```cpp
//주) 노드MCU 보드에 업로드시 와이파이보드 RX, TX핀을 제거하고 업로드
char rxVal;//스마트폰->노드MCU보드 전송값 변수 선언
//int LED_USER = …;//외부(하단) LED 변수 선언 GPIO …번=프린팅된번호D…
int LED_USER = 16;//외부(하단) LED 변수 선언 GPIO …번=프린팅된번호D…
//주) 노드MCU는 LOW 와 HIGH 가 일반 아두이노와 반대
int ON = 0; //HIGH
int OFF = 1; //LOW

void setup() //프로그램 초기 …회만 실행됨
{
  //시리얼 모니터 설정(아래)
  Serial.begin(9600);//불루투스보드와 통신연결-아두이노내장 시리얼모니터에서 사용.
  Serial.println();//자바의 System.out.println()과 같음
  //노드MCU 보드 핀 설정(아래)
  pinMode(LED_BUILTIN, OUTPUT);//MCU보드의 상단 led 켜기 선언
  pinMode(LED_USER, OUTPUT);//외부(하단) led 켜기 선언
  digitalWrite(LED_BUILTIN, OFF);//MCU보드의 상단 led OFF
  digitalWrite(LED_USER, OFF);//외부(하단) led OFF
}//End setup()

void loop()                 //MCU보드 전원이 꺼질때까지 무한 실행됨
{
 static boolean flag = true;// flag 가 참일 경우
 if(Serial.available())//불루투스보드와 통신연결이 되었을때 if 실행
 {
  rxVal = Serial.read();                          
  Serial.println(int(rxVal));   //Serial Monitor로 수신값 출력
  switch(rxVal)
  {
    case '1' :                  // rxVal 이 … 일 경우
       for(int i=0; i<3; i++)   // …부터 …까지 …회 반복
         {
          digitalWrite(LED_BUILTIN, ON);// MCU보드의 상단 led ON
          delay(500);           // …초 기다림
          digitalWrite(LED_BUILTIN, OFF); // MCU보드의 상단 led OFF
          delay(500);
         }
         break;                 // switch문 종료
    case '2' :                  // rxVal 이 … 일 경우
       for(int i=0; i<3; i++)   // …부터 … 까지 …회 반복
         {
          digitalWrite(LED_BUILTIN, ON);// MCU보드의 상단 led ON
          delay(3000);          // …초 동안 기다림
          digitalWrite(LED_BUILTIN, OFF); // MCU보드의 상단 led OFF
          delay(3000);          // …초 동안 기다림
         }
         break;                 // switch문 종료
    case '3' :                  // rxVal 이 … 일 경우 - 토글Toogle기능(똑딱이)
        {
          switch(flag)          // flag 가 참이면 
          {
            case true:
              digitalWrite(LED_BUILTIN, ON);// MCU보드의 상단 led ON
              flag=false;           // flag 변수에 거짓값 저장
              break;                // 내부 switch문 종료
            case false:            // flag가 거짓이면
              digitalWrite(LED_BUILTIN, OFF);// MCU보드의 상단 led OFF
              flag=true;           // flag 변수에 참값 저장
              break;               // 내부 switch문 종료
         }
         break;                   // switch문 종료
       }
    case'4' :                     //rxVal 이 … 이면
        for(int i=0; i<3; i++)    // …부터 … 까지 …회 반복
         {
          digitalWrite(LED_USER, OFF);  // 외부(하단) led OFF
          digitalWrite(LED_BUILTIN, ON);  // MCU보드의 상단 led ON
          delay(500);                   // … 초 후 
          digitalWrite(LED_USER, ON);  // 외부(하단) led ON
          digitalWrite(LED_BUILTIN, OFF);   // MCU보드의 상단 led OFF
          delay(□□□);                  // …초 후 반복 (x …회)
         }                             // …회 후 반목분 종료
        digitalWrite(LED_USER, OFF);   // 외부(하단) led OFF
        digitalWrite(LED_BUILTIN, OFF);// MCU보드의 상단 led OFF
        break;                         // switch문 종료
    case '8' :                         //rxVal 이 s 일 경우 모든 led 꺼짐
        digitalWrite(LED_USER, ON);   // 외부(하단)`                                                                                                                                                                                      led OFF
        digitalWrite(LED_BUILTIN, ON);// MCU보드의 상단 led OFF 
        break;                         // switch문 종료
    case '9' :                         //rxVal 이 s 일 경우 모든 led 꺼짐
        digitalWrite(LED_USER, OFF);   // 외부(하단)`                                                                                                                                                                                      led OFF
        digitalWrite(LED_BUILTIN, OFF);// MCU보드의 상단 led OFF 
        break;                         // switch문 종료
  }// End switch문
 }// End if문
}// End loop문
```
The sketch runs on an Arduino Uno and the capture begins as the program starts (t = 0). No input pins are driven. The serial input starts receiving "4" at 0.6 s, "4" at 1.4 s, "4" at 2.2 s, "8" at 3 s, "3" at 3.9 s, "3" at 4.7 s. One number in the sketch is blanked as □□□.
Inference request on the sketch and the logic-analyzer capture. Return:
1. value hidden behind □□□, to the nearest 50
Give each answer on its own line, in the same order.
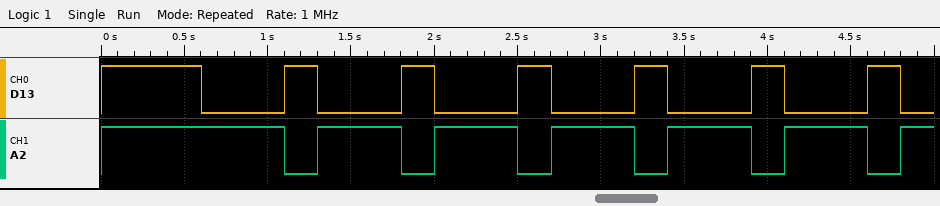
200
